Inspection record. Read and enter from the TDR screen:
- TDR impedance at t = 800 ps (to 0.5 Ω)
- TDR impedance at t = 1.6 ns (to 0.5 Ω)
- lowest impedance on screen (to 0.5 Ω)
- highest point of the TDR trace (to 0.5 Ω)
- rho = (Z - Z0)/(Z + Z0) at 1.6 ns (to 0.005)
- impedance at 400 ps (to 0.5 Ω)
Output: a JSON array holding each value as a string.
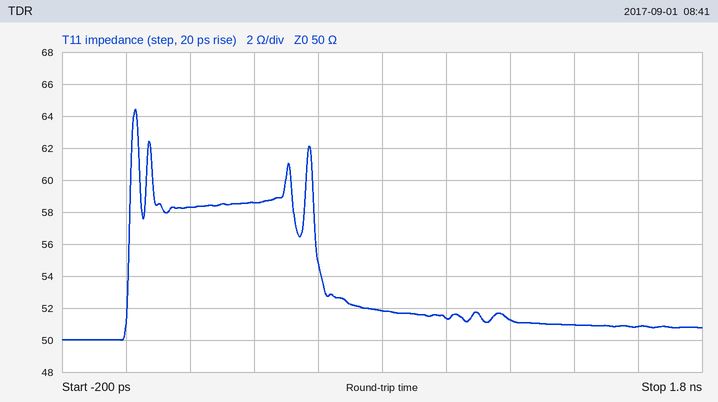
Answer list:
["52.0 Ω", "51.0 Ω", "50.0 Ω", "64.5 Ω", "+0.010", "58.5 Ω"]
